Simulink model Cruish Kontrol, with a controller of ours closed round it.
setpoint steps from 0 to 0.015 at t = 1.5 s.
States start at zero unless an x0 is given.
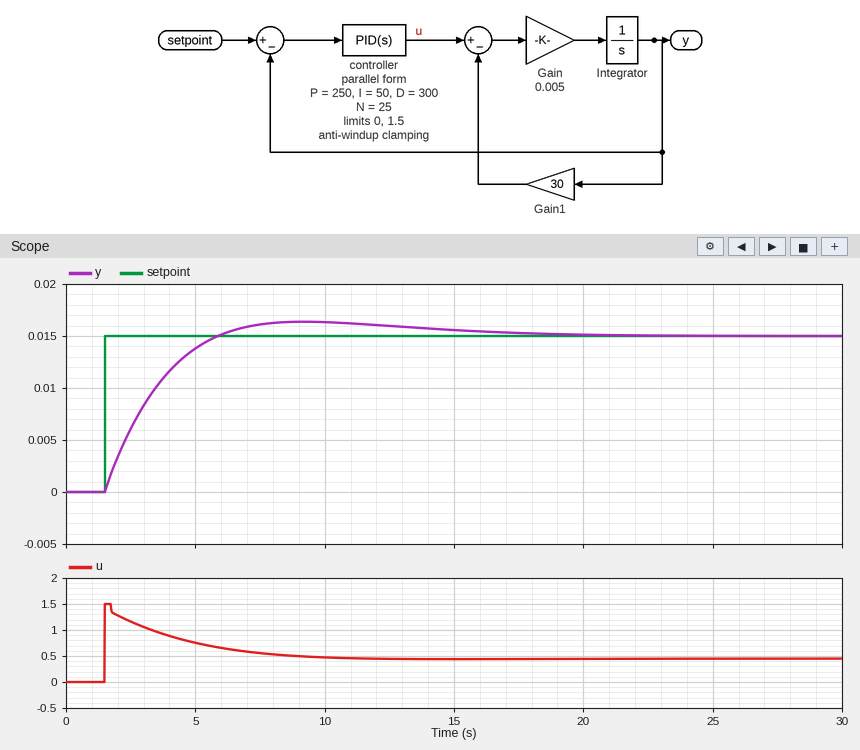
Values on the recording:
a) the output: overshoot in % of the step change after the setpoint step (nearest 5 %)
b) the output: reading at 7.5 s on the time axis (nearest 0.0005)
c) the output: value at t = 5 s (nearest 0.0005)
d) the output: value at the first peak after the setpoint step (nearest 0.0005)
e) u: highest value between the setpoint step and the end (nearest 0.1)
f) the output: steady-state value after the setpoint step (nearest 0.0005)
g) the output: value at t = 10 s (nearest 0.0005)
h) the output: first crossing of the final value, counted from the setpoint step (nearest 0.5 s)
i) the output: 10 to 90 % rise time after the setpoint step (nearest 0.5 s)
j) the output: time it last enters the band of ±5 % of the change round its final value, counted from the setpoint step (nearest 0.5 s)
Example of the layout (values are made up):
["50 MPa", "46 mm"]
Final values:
["10 %", "0.0160", "0.0140", "0.0165", "1.5", "0.0150", "0.0165", "4.5 s", "3.0 s", "12.5 s"]
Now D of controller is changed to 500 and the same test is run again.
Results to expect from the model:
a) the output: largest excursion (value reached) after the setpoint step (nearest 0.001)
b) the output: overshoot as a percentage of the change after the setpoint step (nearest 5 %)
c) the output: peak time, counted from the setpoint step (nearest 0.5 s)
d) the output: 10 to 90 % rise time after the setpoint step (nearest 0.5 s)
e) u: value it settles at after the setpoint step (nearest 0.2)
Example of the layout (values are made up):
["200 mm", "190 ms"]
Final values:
["0.017", "15 %", "9.0 s", "4.0 s", "0.4"]
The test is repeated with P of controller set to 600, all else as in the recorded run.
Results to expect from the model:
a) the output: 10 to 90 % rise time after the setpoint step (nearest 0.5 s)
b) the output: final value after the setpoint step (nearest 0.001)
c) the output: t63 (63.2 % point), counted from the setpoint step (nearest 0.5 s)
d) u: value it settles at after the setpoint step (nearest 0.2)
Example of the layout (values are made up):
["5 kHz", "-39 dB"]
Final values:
["2.5 s", "0.015", "1.5 s", "0.4"]
